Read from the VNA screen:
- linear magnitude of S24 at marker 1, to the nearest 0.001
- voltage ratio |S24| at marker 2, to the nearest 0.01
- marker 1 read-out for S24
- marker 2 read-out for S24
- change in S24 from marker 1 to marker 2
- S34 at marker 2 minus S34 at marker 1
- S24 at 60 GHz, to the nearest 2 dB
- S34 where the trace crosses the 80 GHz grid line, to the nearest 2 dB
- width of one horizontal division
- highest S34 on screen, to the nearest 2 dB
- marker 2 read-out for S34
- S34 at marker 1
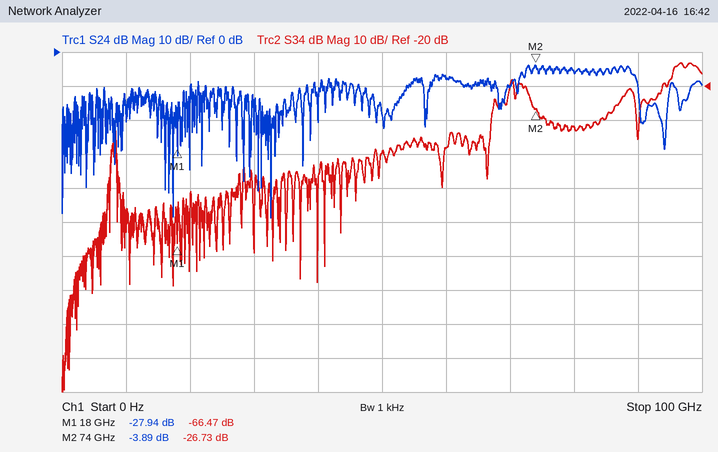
0.040
0.64
-27.94 dB
-3.89 dB
24.05 dB
39.74 dB
-8 dB
-32 dB
10 GHz
-14 dB
-26.73 dB
-66.47 dB
